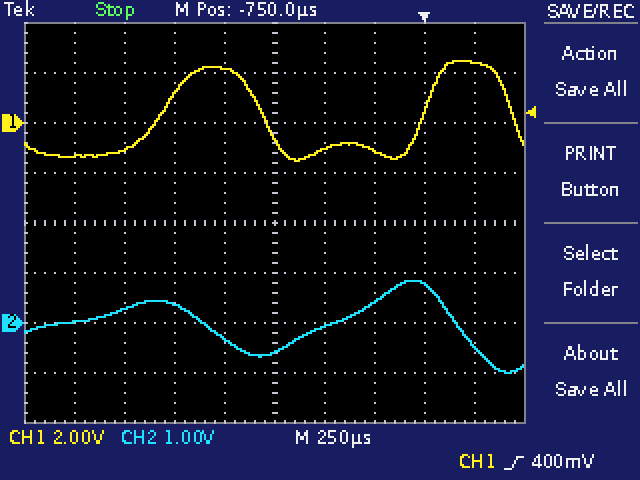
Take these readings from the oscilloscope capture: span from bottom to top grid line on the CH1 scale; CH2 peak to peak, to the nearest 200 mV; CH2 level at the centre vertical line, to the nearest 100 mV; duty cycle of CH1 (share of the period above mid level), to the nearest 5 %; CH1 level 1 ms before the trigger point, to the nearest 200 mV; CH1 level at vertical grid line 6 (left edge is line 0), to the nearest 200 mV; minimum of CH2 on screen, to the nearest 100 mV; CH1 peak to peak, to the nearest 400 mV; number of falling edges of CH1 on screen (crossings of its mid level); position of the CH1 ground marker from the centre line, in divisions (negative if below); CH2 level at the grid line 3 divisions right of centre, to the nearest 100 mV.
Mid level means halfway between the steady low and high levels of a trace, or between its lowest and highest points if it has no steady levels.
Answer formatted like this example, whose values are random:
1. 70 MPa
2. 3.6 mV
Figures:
1. 16 V
2. 1.8 V
3. -600 mV
4. 35 %
5. 2.2 V
6. -1.0 V
7. -1.0 V
8. 4.0 V
9. 2
10. +2.0 div
11. 800 mV
